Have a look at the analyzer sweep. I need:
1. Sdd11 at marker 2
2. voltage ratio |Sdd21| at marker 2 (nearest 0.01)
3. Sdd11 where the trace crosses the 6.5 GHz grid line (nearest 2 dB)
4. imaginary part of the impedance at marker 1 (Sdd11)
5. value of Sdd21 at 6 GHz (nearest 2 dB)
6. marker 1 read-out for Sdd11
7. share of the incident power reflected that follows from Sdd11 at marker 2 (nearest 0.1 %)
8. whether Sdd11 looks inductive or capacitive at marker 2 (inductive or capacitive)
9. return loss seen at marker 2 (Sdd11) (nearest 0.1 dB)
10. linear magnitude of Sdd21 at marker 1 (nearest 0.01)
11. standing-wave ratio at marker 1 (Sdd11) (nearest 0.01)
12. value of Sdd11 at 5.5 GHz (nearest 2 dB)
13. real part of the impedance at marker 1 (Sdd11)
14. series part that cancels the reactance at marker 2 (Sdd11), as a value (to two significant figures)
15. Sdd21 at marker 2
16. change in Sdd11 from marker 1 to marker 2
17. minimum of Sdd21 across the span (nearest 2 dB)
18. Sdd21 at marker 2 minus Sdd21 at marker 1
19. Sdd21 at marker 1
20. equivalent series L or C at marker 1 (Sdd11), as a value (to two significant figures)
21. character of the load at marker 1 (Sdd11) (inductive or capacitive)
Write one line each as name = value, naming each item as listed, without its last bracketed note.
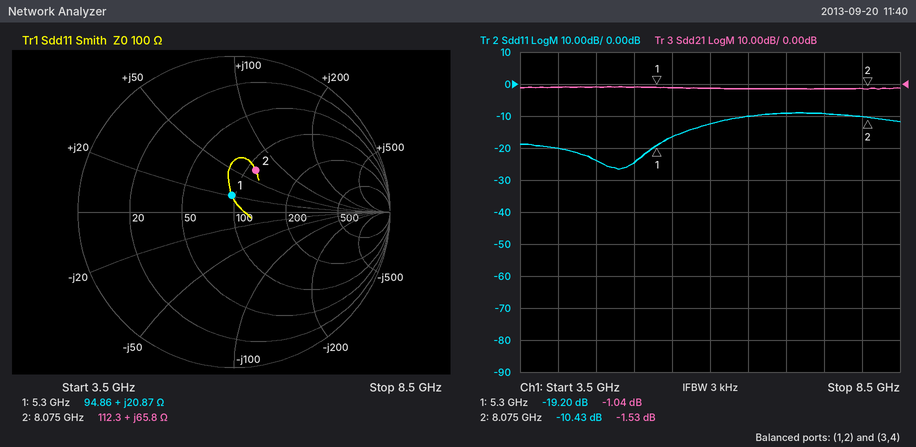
Sdd11 at marker 2 = -10.43 dB
voltage ratio |Sdd21| at marker 2 = 0.84
Sdd11 where the trace crosses the 6.5 GHz grid line = -10 dB
imaginary part of the impedance at marker 1 = +20.87 Ω
value of Sdd21 at 6 GHz = -2 dB
marker 1 read-out for Sdd11 = -19.20 dB
share of the incident power reflected that follows from Sdd11 at marker 2 = 9.1 %
whether Sdd11 looks inductive or capacitive at marker 2 = inductive
return loss seen at marker 2 (Sdd11) = 10.4 dB
linear magnitude of Sdd21 at marker 1 = 0.89
standing-wave ratio at marker 1 (Sdd11) = 1.25
value of Sdd11 at 5.5 GHz = -16 dB
real part of the impedance at marker 1 = 94.86 Ω
series part that cancels the reactance at marker 2 (Sdd11), as a value = 300 fF
Sdd21 at marker 2 = -1.53 dB
change in Sdd11 from marker 1 to marker 2 = 8.77 dB
minimum of Sdd21 across the span = -2 dB
Sdd21 at marker 2 minus Sdd21 at marker 1 = -0.49 dB
Sdd21 at marker 1 = -1.04 dB
equivalent series L or C at marker 1 (Sdd11), as a value = 630 pH
character of the load at marker 1 (Sdd11) = inductive
